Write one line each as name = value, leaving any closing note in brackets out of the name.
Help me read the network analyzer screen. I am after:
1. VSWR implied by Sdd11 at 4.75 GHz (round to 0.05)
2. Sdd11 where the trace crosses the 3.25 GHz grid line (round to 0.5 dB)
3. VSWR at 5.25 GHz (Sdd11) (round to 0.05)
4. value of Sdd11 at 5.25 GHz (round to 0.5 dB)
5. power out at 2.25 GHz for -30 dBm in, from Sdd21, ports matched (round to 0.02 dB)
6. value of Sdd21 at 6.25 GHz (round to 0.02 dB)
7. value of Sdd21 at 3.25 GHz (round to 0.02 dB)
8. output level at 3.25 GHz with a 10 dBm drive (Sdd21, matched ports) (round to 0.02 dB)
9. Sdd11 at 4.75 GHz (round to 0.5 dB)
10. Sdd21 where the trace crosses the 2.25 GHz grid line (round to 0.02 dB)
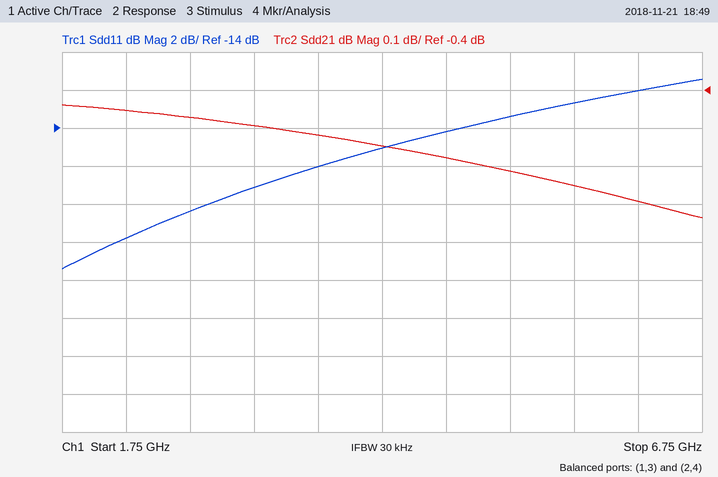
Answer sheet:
VSWR implied by Sdd11 at 4.75 GHz = 1.50
Sdd11 where the trace crosses the 3.25 GHz grid line = -17.0 dB
VSWR at 5.25 GHz (Sdd11) = 1.55
value of Sdd11 at 5.25 GHz = -13.5 dB
power out at 2.25 GHz for -30 dBm in, from Sdd21, ports matched = -30.46 dBm
value of Sdd21 at 6.25 GHz = -0.70 dB
value of Sdd21 at 3.25 GHz = -0.50 dB
output level at 3.25 GHz with a 10 dBm drive (Sdd21, matched ports) = 9.50 dBm
Sdd11 at 4.75 GHz = -14.0 dB
Sdd21 where the trace crosses the 2.25 GHz grid line = -0.46 dB
